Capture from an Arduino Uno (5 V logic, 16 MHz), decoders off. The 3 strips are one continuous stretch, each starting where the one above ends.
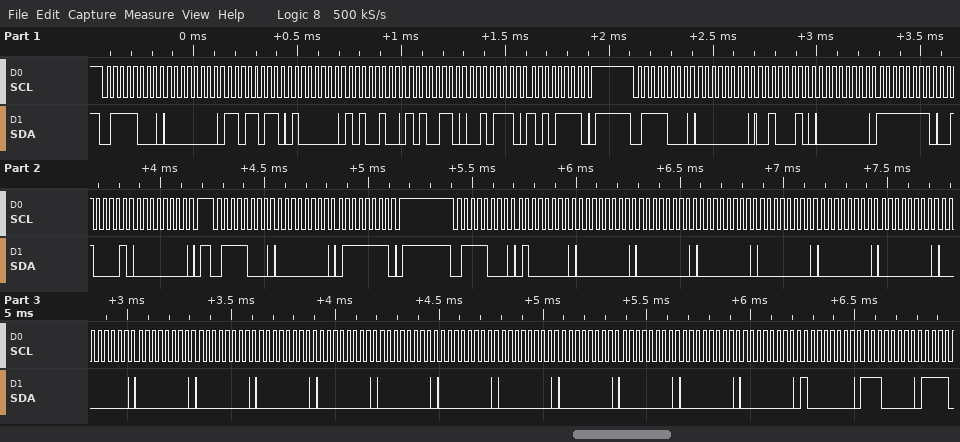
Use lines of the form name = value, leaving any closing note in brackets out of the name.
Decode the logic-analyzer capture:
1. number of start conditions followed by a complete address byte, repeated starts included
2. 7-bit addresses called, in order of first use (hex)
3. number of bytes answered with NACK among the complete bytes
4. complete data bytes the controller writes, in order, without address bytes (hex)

number of start conditions followed by a complete address byte, repeated starts included = 4
7-bit addresses called, in order of first use = 0x3C
number of bytes answered with NACK among the complete bytes = 0
complete data bytes the controller writes, in order, without address bytes = 00 DB 40 A4 A6 2E AF 00 22 00 FF 21 00 00 7F 40 00 00 00 00 00 00 00 00 00 00 00 00 00 00 00 00 00 00 80 E0
